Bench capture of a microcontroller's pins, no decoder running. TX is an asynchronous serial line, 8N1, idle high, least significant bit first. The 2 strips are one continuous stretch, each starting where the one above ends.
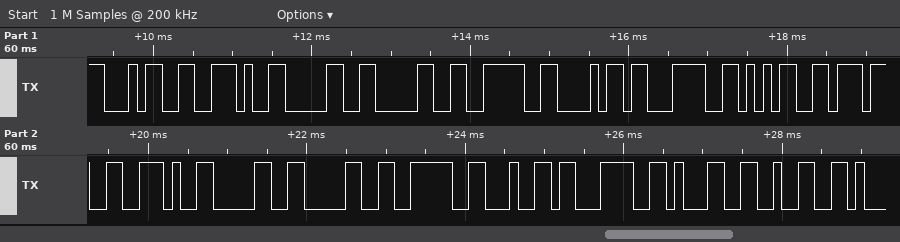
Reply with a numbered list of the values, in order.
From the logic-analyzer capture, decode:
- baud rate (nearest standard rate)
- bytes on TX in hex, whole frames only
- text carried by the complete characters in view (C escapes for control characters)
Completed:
1. 9600 baud
2. 34 2E 30 30 3E 68 3C 35 37 2E 30 30 3E 64 3C 31 32
3. "4.00>h<57.00>d<12"
